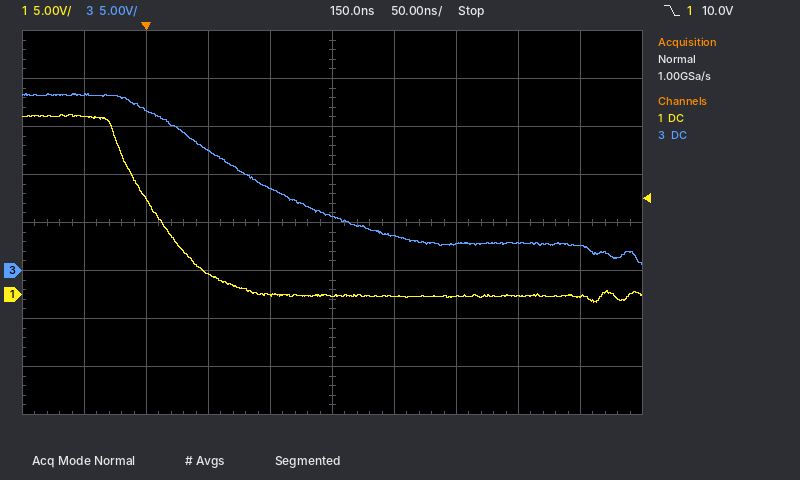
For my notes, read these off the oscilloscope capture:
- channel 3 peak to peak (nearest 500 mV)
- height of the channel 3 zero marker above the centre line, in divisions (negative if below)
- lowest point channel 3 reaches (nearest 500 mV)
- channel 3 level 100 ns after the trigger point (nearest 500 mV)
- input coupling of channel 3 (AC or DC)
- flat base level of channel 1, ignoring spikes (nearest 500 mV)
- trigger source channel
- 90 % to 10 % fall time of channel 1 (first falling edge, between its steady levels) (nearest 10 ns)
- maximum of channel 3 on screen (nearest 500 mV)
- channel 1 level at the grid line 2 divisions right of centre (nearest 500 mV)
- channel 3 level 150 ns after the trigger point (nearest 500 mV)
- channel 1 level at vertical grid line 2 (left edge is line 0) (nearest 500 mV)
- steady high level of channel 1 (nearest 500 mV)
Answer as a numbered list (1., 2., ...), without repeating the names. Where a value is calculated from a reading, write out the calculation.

1. 18.5 V − (500 mV) = 18.0 V
2. -1.0 div
3. 500 mV
4. 8.5 V
5. DC
6. 0.0 V
7. channel 1
8. 80 ns
9. 18.5 V
10. 0.0 V
11. 5.5 V
12. 10.0 V
13. 18.5 V
